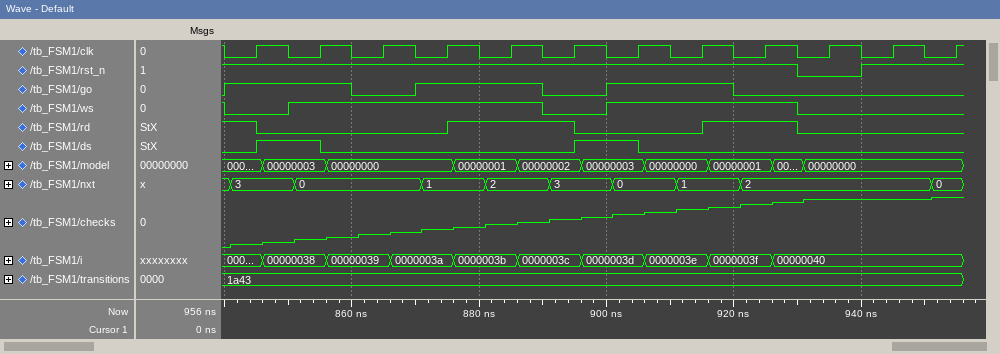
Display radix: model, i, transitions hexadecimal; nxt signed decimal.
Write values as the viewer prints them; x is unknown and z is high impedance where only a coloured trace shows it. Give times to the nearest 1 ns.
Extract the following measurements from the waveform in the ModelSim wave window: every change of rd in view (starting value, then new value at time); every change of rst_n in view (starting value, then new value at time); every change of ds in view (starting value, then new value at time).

1, 0 at 845 ns, 1 at 875 ns, 0 at 895 ns, 1 at 915 ns, 0 at 930 ns
1, 0 at 930 ns, 1 at 940 ns
0, 1 at 845 ns, 0 at 855 ns, 1 at 895 ns, 0 at 905 ns
